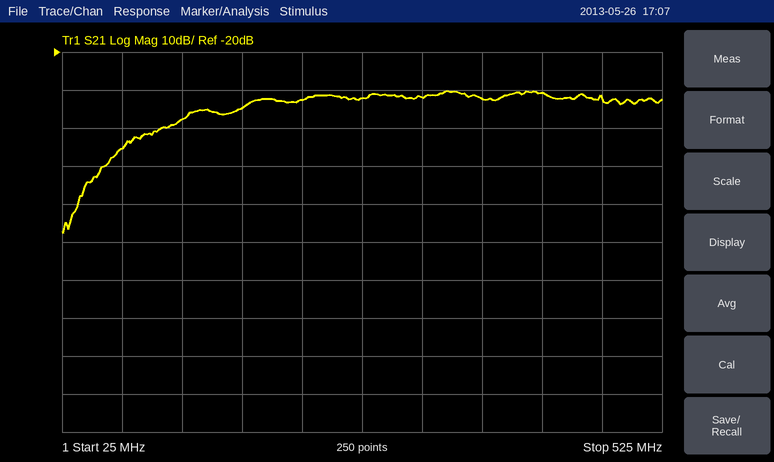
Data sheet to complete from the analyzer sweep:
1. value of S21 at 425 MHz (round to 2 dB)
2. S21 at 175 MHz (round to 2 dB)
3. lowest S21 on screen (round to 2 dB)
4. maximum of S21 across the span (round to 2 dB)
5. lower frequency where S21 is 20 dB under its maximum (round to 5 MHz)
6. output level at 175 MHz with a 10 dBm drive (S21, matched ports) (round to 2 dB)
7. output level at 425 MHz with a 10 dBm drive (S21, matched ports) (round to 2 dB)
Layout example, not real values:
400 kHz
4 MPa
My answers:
-30 dB
-34 dB
-68 dB
-30 dB
60 MHz
-24 dBm
-20 dBm
